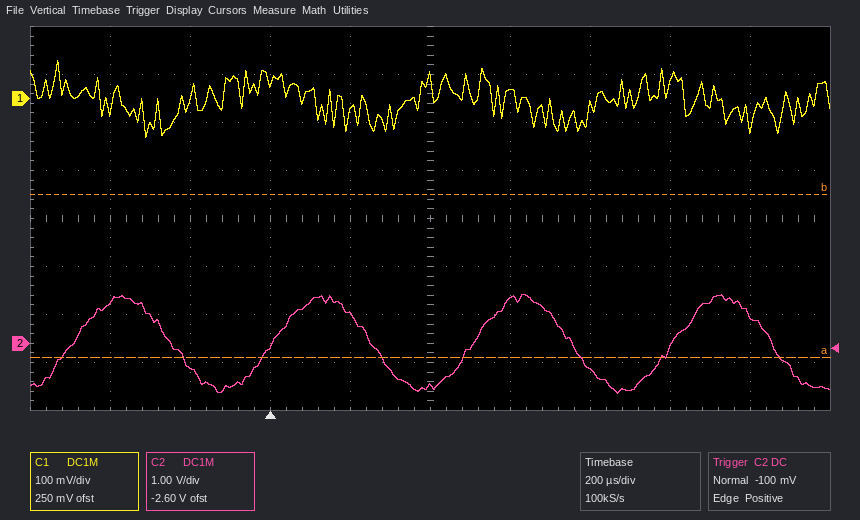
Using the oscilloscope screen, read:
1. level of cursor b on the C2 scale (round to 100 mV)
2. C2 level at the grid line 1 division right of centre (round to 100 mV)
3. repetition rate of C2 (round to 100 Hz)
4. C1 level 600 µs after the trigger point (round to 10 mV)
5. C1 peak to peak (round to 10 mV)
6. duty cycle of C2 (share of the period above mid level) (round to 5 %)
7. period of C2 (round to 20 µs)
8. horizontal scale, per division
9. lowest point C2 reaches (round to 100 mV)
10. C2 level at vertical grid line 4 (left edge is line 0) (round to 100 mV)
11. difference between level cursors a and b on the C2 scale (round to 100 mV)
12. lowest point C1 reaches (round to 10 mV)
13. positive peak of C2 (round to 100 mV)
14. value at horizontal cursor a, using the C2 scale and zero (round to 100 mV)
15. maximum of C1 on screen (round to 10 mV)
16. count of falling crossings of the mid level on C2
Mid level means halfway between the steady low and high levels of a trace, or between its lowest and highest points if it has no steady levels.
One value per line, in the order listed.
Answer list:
3.1 V
900 mV
2.0 kHz
20 mV
160 mV
50 %
500 µs
200 µs
-1.0 V
600 mV
3.4 V
-80 mV
1.0 V
-300 mV
80 mV
4
